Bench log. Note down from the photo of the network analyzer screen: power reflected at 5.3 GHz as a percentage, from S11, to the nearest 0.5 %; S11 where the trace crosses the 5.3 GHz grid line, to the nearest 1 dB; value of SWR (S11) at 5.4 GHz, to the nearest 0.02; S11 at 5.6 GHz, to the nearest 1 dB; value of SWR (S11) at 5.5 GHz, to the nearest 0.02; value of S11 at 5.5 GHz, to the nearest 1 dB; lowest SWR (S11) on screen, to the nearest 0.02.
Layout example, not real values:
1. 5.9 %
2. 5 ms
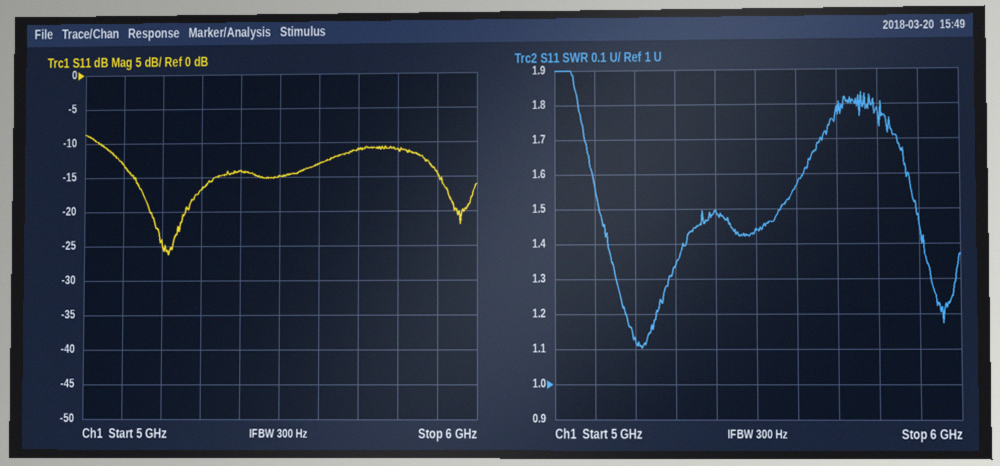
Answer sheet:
1. 2.0 %
2. -17 dB
3. 1.50
4. -13 dB
5. 1.44
6. -15 dB
7. 1.10
